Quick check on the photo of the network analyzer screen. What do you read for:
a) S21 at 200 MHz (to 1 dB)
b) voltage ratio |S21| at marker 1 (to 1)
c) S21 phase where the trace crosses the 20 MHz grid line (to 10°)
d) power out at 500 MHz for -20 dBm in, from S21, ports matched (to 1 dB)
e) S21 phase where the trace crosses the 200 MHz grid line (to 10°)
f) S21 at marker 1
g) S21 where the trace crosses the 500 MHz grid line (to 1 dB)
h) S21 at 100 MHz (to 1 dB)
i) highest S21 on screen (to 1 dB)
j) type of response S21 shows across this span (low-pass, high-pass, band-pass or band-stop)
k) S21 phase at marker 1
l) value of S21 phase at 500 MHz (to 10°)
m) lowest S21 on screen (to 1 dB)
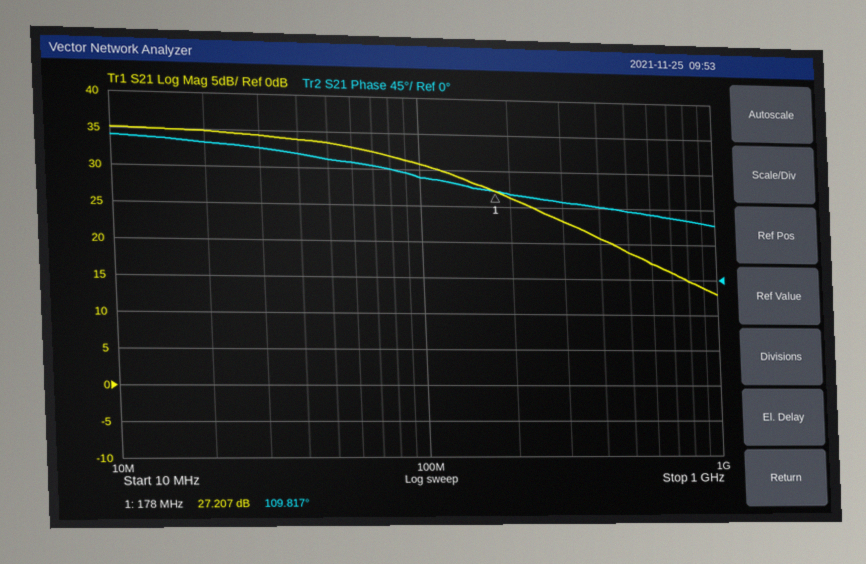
26 dB
23
160°
-1 dBm
110°
27.207 dB
19 dB
31 dB
35 dB
low-pass
109.817°
90°
13 dB
